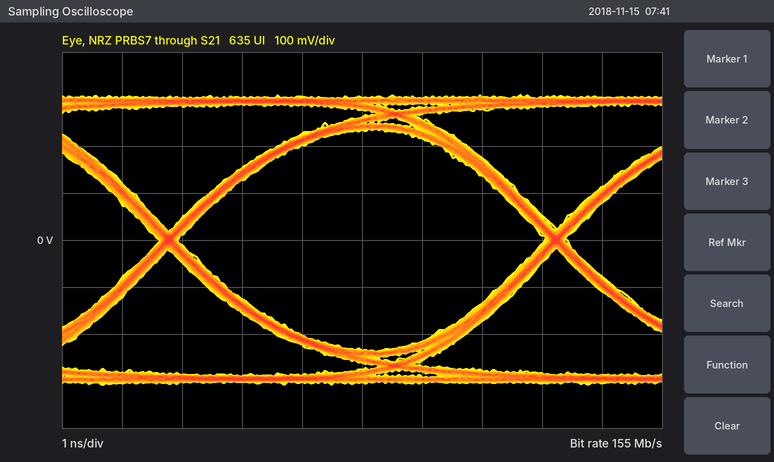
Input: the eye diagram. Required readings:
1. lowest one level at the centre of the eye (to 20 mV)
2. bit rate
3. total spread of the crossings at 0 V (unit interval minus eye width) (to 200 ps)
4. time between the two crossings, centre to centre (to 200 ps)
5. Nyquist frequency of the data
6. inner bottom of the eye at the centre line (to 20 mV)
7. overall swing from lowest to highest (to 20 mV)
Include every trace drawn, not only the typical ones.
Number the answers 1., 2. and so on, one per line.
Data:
1. 240 mV
2. 155 Mb/s
3. 400 ps
4. 6.4 ns
5. 77.5 MHz
6. -240 mV
7. 620 mV
